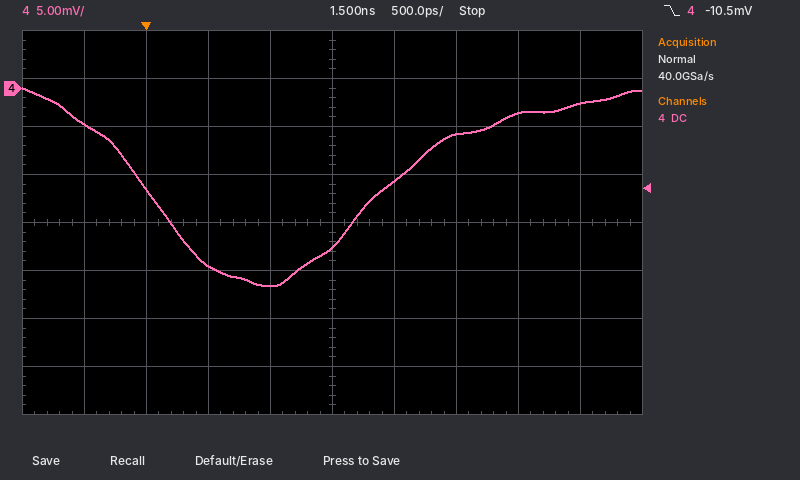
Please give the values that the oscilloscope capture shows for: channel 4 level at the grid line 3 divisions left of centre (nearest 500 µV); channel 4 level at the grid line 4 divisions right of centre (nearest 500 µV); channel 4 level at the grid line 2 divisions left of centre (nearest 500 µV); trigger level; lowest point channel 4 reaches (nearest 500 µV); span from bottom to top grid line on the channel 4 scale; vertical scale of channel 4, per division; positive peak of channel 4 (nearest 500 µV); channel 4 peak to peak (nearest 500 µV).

-10.5 mV
-1.5 mV
-18.5 mV
-10.5 mV
-20.5 mV
40 mV
5 mV
0.0 mV
20.5 mV
